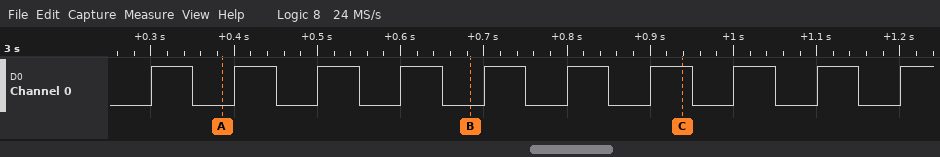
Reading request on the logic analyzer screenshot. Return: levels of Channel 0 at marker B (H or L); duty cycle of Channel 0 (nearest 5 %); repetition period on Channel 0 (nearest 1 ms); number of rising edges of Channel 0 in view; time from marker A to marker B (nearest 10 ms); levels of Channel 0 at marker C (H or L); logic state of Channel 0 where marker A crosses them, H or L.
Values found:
Channel 0=L
50 %
100 ms
10
300 ms
Channel 0=H
Channel 0=L
